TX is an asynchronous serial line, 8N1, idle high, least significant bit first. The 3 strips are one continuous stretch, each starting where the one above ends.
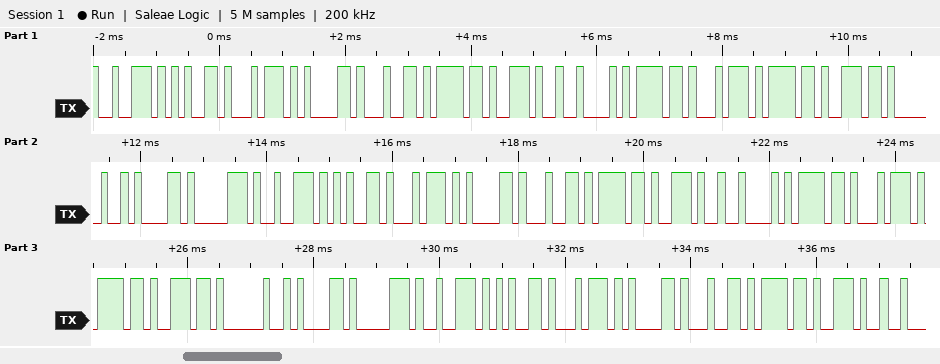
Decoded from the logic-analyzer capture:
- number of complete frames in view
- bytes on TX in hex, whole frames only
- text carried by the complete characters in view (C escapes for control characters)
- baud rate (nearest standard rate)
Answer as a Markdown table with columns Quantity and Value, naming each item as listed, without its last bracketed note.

| Quantity | Value |
|---|---|
| number of complete frames in view | 37 |
| bytes on TX in hex, whole frames only | 72 65 74 61 64 6F 2E 42 6F 74 6F 6E 20 61 70 72 65 74 61 64 6F 2E 42 6F 74 6F 6E 20 61 70 72 65 74 61 64 6F 2E |
| text carried by the complete characters in view | "retado.Boton apretado.Boton apretado." |
| baud rate | 9600 baud |
